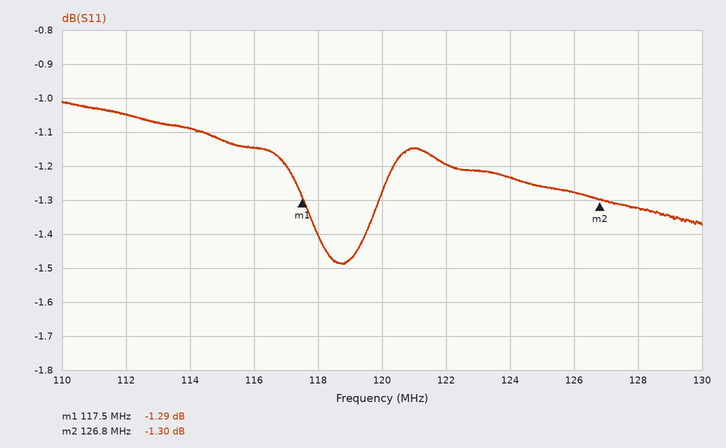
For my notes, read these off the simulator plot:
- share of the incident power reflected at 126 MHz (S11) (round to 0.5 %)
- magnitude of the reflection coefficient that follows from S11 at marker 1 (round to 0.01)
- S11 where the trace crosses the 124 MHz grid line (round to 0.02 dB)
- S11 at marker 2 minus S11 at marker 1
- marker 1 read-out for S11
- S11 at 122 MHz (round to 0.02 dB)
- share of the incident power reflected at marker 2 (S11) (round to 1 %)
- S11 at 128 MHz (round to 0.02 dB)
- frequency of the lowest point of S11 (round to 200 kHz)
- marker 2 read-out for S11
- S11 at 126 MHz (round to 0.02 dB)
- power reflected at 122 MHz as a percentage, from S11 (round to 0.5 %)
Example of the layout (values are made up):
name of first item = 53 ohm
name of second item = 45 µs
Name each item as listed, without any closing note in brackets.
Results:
share of the incident power reflected at 126 MHz (S11) = 74.5 %
magnitude of the reflection coefficient that follows from S11 at marker 1 = 0.86
S11 where the trace crosses the 124 MHz grid line = -1.24 dB
S11 at marker 2 minus S11 at marker 1 = -0.01 dB
marker 1 read-out for S11 = -1.29 dB
S11 at 122 MHz = -1.20 dB
share of the incident power reflected at marker 2 (S11) = 74 %
S11 at 128 MHz = -1.32 dB
frequency of the lowest point of S11 = 118.8 MHz
marker 2 read-out for S11 = -1.30 dB
S11 at 126 MHz = -1.28 dB
power reflected at 122 MHz as a percentage, from S11 = 76.0 %
